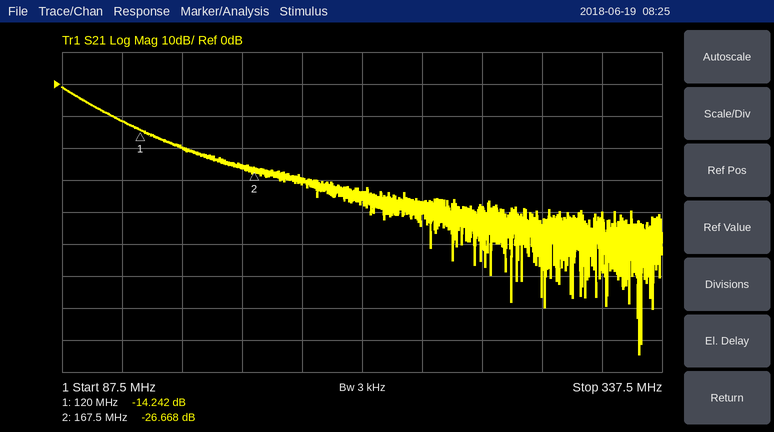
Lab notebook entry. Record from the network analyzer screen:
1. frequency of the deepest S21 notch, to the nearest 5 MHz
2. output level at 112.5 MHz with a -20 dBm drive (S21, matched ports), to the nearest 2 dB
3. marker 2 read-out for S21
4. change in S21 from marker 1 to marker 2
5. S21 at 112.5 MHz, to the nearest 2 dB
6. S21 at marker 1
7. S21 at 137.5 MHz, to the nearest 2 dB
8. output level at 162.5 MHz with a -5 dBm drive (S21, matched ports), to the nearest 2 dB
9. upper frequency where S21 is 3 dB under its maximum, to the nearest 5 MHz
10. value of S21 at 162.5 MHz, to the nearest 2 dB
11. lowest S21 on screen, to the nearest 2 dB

330 MHz
-32 dBm
-26.668 dB
-12.426 dB
-12 dB
-14.242 dB
-20 dB
-30 dBm
95 MHz
-26 dB
-84 dB
